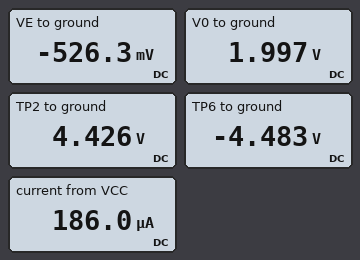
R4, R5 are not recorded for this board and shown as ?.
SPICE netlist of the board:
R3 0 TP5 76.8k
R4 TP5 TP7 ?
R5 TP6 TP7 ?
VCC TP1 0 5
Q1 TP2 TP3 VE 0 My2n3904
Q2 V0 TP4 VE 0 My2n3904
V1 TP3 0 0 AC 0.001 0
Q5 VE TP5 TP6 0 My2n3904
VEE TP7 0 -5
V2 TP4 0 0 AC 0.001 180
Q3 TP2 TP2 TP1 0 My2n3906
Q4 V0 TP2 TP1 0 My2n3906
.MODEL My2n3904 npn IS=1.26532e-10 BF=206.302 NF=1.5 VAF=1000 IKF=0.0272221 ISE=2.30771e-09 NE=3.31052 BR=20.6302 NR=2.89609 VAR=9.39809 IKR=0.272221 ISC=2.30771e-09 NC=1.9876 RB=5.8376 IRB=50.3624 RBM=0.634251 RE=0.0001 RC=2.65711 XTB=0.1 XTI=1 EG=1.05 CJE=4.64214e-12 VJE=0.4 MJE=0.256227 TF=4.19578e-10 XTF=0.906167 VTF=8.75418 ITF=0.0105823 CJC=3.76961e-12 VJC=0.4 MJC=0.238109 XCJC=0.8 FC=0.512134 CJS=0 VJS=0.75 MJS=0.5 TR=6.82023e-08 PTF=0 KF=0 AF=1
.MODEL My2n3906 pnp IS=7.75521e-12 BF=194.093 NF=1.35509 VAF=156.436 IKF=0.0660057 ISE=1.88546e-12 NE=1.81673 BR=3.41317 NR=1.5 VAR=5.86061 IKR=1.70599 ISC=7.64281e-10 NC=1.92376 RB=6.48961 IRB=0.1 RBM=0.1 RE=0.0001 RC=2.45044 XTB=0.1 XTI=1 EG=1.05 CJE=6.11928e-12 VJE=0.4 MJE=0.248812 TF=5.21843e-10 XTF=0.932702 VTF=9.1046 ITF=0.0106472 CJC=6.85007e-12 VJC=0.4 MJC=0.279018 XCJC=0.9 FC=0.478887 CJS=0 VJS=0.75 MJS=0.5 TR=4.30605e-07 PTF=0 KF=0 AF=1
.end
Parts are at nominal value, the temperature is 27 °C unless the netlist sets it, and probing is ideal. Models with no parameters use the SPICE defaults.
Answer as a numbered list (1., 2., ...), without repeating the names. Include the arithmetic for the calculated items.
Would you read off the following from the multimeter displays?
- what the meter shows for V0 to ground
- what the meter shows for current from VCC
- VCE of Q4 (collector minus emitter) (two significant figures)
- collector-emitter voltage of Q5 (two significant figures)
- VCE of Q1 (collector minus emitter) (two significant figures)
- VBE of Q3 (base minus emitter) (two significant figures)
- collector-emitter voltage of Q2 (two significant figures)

1. 1.997 V
2. 186.0 µA
3. 1.997 V - 5 V = -3.0 V
4. -526.3 mV - (-4.483 V) = 4.0 V
5. 4.426 V - (-526.3 mV) = 5.0 V
6. 4.426 V - 5 V = -570 mV
7. 1.997 V - (-526.3 mV) = 2.5 V
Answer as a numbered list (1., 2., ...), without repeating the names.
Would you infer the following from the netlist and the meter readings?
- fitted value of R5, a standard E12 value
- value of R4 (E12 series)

1. 2.7 kΩ
2. 22 kΩ
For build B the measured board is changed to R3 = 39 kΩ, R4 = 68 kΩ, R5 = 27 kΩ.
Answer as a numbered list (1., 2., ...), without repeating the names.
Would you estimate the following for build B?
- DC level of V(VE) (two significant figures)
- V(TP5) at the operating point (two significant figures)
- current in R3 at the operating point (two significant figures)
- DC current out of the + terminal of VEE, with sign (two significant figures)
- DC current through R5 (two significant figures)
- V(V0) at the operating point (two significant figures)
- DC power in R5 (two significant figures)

1. -500 mV
2. -1.9 V
3. 48 µA
4. -140 µA
5. 97 µA
6. 1.8 V
7. 250 µW
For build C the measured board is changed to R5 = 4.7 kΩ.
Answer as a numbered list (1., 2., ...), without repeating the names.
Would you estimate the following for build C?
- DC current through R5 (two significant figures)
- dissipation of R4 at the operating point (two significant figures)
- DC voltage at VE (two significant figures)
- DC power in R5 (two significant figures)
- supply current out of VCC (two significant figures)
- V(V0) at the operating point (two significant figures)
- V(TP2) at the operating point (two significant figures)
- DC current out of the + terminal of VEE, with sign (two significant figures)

1. 120 µA
2. 53 µW
3. -510 mV
4. 64 µW
5. 110 µA
6. 1.9 V
7. 4.4 V
8. -170 µA
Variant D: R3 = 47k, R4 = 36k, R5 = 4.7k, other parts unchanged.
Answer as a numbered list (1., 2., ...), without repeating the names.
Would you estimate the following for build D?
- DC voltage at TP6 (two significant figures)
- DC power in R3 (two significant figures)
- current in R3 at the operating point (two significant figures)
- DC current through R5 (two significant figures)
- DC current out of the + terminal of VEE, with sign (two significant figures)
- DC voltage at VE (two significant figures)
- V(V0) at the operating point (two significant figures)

1. -3.5 V
2. 180 µW
3. 62 µA
4. 320 µA
5. -380 µA
6. -550 mV
7. 2.1 V
